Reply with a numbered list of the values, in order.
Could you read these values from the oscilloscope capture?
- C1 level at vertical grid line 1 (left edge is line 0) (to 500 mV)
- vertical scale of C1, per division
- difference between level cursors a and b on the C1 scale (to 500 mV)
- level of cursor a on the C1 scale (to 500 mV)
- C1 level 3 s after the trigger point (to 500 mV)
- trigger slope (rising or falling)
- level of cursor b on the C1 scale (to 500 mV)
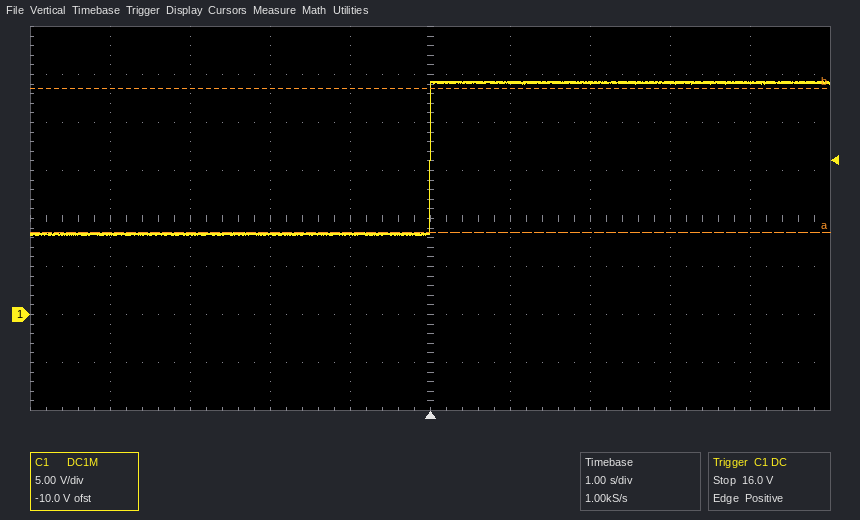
1. 8.5 V
2. 5 V
3. 15.0 V
4. 8.5 V
5. 24.0 V
6. rising
7. 23.5 V
